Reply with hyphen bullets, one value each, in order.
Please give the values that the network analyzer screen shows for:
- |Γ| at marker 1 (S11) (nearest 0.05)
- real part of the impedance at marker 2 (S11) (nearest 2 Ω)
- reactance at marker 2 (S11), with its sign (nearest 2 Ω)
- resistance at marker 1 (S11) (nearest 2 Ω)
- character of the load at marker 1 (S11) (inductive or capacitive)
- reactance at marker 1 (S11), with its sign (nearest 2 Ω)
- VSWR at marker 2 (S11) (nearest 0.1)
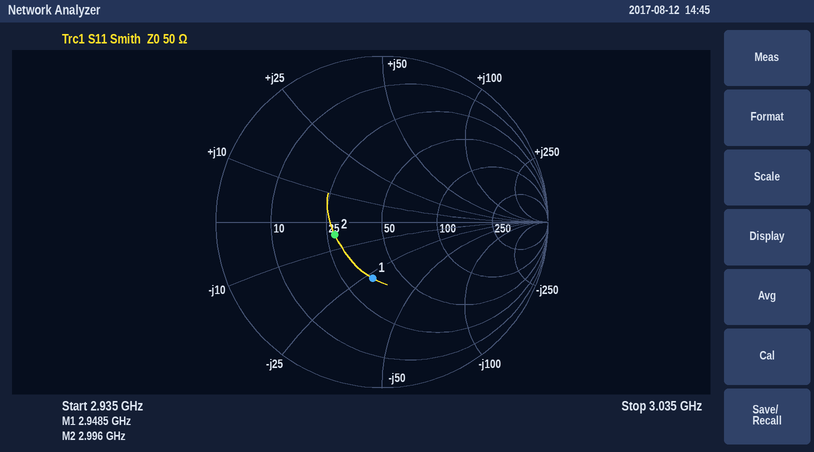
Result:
- 0.35
- 28 Ω
- -4 Ω
- 36 Ω
- capacitive
- -28 Ω
- 1.8
